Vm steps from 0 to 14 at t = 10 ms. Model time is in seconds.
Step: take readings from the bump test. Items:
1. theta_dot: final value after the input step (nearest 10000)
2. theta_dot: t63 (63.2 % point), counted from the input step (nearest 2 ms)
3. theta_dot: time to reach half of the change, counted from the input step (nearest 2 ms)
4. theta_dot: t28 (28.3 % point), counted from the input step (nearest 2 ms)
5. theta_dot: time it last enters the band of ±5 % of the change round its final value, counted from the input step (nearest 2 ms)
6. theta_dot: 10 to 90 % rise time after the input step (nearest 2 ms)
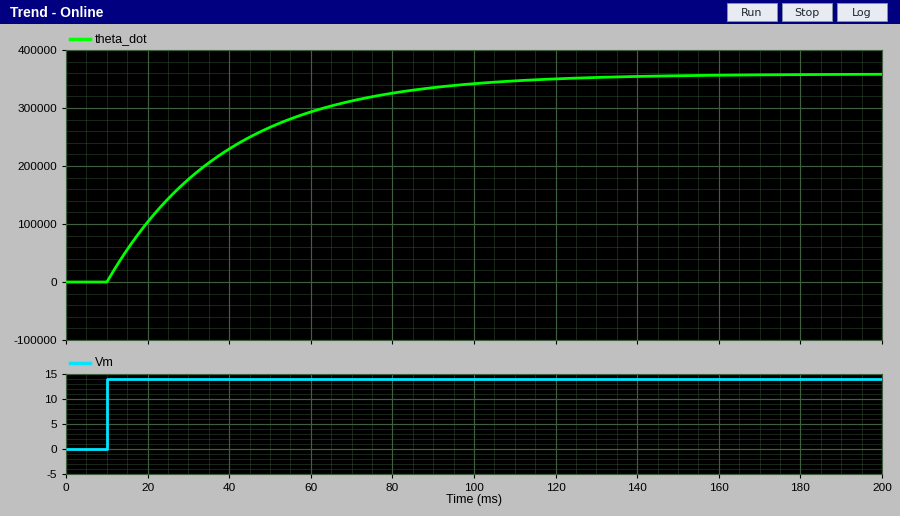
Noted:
360000
30 ms
20 ms
10 ms
88 ms
64 ms
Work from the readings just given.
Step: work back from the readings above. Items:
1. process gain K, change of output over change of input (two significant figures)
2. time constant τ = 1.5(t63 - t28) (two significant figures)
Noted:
26000
30 ms
